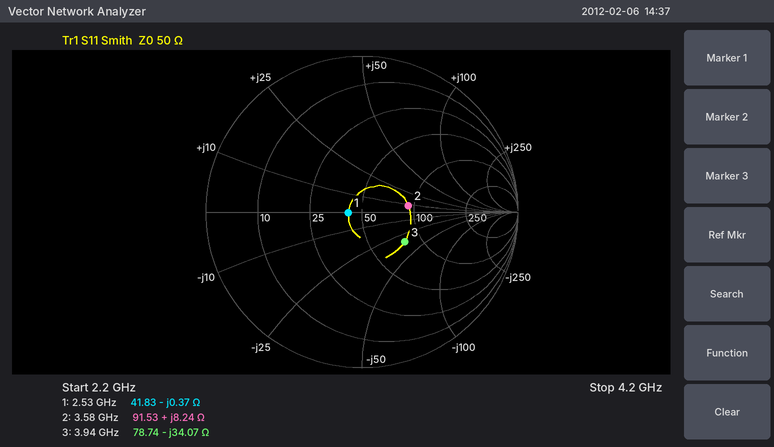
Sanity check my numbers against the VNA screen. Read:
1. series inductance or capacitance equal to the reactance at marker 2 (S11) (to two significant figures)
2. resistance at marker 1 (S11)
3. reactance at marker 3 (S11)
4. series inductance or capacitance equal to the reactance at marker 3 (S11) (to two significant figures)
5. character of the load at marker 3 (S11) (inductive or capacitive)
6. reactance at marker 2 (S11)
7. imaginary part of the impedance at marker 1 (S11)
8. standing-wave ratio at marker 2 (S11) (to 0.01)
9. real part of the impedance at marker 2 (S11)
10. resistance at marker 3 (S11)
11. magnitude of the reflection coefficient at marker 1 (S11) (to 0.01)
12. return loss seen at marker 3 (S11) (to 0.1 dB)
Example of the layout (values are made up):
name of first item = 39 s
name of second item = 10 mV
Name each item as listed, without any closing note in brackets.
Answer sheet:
series inductance or capacitance equal to the reactance at marker 2 (S11) = 370 pH
resistance at marker 1 = 41.83 Ω
reactance at marker 3 = -34.07 Ω
series inductance or capacitance equal to the reactance at marker 3 (S11) = 1.2 pF
character of the load at marker 3 (S11) = capacitive
reactance at marker 2 = +8.24 Ω
imaginary part of the impedance at marker 1 = -0.37 Ω
standing-wave ratio at marker 2 (S11) = 1.85
real part of the impedance at marker 2 = 91.53 Ω
resistance at marker 3 = 78.74 Ω
magnitude of the reflection coefficient at marker 1 (S11) = 0.09
return loss seen at marker 3 (S11) = 9.5 dB
